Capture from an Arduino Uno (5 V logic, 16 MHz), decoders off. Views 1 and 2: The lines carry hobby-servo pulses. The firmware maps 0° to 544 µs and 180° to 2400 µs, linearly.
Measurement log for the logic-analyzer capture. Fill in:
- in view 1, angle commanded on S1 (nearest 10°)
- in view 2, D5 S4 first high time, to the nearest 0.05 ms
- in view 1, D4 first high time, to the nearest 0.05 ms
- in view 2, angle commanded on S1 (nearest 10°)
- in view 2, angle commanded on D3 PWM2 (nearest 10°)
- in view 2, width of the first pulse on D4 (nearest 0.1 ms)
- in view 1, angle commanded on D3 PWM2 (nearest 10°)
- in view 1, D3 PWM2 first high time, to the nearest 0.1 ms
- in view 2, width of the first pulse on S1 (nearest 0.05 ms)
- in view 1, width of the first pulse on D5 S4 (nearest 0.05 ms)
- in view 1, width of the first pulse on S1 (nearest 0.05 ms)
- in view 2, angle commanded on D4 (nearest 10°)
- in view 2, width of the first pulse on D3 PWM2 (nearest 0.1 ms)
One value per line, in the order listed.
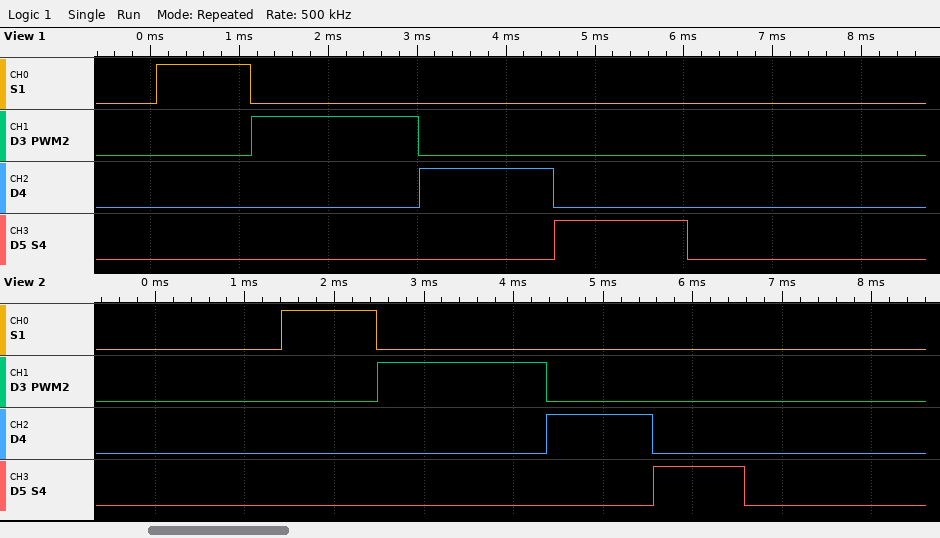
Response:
50°
1.00 ms
1.50 ms
50°
130°
1.2 ms
130°
1.9 ms
1.05 ms
1.50 ms
1.05 ms
60°
1.9 ms
